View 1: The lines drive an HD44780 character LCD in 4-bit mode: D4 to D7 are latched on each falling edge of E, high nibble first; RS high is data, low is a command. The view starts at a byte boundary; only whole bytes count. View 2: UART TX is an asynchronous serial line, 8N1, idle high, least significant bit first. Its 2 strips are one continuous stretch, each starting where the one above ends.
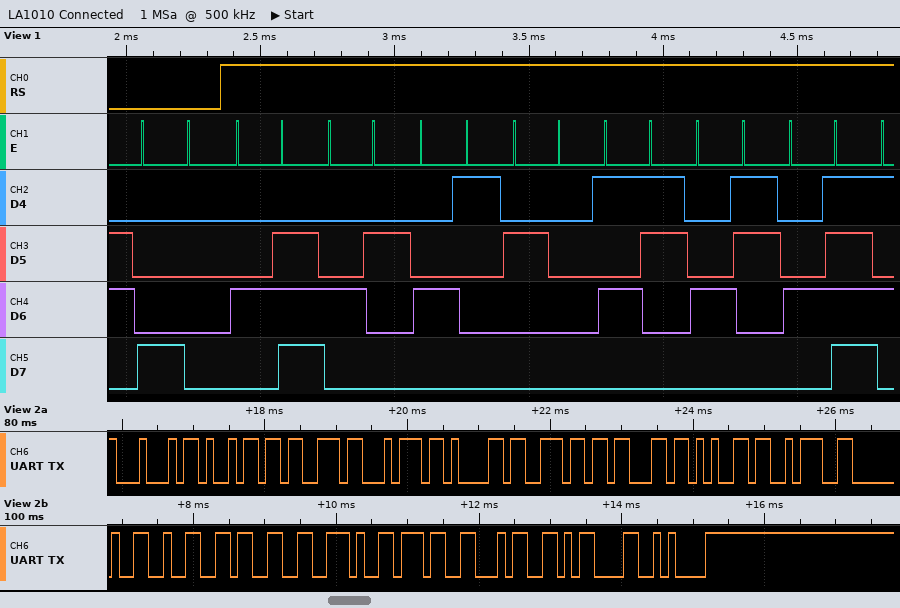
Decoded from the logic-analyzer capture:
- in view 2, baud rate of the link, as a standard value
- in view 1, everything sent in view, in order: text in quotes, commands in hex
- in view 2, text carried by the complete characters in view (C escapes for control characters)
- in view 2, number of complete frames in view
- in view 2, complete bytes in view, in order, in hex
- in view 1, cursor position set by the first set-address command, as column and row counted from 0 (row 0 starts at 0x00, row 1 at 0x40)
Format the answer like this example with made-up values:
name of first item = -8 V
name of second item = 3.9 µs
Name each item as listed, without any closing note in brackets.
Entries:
in view 2, baud rate of the link, as a standard value = 9600 baud
in view 1, everything sent in view, in order: text in quotes, commands in hex = 0x80 "NBA SCO"
in view 2, text carried by the complete characters in view = "Distance: 23.74\r\n"
in view 2, number of complete frames in view = 17
in view 2, complete bytes in view, in order, in hex = 44 69 73 74 61 6E 63 65 3A 20 32 33 2E 37 34 0D 0A
in view 1, cursor position set by the first set-address command, as column and row counted from 0 = column 0, row 0
